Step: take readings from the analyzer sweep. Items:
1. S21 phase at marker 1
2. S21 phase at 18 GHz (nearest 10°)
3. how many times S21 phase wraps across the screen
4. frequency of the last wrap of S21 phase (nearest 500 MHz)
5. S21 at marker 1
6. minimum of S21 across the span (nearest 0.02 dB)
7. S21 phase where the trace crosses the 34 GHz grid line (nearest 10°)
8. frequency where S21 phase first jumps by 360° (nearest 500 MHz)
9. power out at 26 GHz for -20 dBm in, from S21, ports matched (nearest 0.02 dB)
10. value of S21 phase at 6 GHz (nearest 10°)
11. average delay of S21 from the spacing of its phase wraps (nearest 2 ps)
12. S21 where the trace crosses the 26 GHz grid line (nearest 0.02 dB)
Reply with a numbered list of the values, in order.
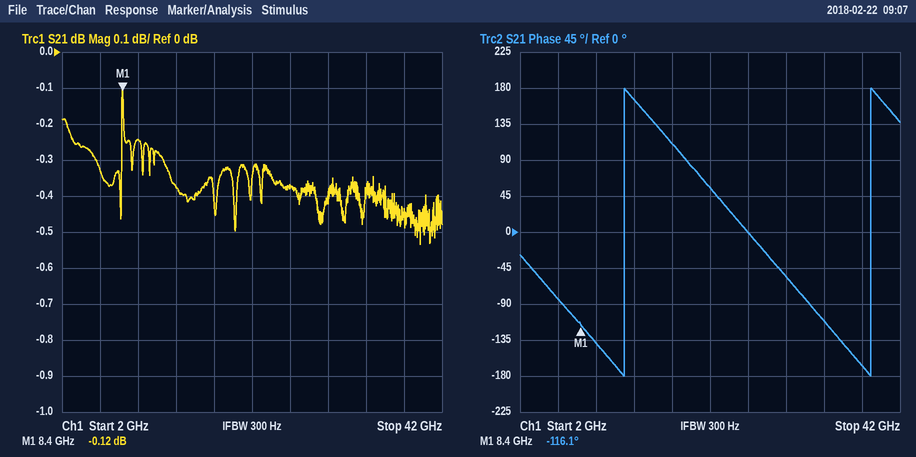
1. -116.1°
2. 110°
3. 2
4. 39.0 GHz
5. -0.12 dB
6. -0.54 dB
7. -110°
8. 13.0 GHz
9. -20.38 dBm
10. -80°
11. 38 ps
12. -0.38 dB
